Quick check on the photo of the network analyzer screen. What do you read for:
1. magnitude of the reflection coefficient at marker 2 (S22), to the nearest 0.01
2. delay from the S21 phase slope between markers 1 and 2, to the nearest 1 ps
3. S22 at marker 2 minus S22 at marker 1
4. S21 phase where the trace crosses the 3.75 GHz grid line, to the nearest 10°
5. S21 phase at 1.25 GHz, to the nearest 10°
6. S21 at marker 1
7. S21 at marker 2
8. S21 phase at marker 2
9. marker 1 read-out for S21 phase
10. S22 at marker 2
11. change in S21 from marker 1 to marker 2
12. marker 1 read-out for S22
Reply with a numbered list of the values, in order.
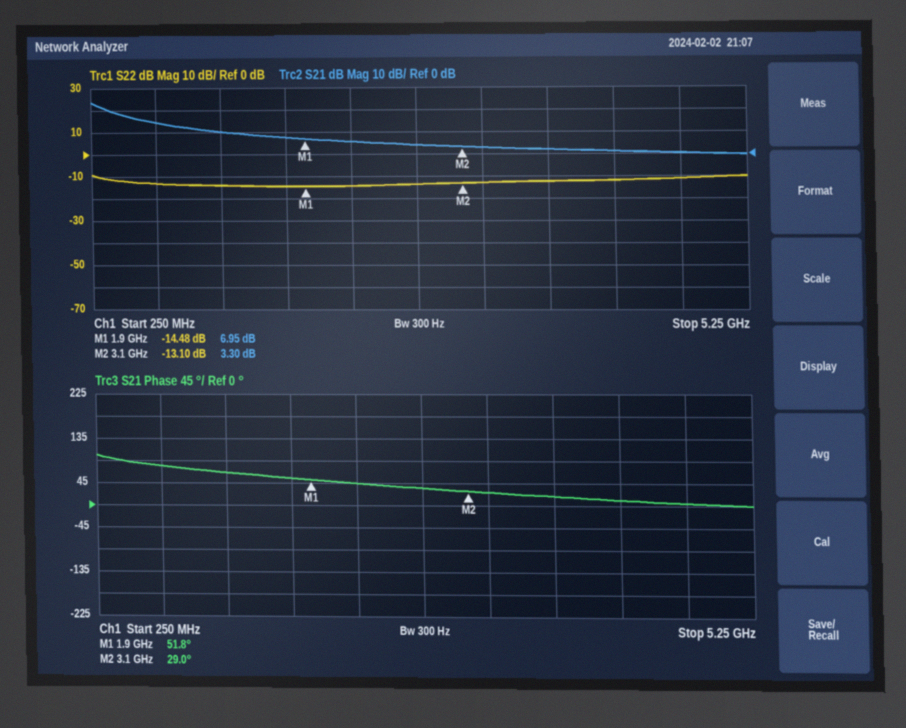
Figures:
1. 0.22
2. 53 ps
3. 1.38 dB
4. 20°
5. 70°
6. 6.95 dB
7. 3.30 dB
8. 29.0°
9. 51.8°
10. -13.10 dB
11. -3.65 dB
12. -14.48 dB
